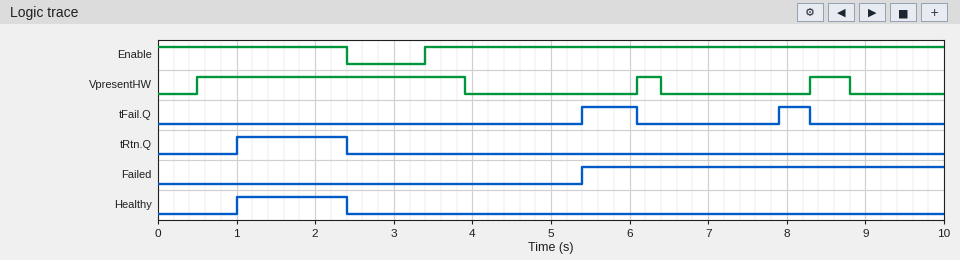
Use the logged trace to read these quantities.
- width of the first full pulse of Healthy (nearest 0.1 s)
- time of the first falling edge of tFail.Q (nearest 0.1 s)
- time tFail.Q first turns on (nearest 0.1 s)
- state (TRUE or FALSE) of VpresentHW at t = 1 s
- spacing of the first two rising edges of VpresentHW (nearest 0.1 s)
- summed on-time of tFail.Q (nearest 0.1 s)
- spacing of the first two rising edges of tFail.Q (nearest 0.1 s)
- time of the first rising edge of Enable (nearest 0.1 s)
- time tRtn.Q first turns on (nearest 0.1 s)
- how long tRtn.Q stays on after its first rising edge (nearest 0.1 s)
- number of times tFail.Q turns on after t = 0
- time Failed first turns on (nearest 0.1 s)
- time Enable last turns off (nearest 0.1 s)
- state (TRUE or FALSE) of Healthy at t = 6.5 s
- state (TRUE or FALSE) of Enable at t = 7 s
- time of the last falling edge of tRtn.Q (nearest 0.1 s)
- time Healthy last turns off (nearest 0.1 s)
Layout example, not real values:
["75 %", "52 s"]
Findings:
["1.4 s", "6.1 s", "5.4 s", "TRUE", "5.6 s", "1.1 s", "2.5 s", "3.4 s", "1.0 s", "1.4 s", "2", "5.4 s", "2.4 s", "FALSE", "TRUE", "2.4 s", "2.4 s"]
